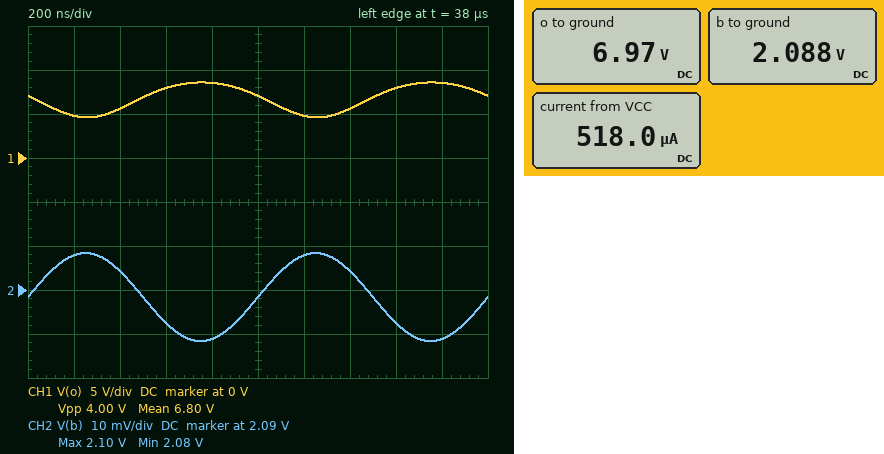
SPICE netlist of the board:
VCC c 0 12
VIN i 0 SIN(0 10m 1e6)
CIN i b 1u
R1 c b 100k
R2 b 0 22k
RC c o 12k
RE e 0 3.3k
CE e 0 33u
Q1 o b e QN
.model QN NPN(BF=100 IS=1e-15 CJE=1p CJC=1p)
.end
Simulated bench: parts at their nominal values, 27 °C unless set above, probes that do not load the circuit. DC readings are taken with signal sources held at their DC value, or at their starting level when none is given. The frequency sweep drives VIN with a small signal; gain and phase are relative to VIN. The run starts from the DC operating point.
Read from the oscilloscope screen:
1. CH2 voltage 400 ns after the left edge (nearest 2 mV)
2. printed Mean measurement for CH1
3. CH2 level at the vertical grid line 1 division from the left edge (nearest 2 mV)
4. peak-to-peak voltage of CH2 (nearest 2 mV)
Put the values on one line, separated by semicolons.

2.094 V; 6.80 V; 2.098 V; 20 mV
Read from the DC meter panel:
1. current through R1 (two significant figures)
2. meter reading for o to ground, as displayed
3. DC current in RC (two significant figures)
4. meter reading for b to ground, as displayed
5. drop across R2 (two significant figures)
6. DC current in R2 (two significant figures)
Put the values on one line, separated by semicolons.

99 µA; 6.97 V; 420 µA; 2.088 V; 2.1 V; 95 µA
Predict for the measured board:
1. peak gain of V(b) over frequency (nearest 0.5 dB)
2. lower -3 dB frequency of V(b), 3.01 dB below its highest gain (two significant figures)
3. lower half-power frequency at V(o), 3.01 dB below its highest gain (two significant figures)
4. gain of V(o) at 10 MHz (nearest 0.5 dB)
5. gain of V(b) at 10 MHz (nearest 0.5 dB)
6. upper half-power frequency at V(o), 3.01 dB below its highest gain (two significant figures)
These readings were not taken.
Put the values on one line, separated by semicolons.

0 dB; 19 Hz; 110 Hz; 45.0 dB; 0 dB; 26 MHz
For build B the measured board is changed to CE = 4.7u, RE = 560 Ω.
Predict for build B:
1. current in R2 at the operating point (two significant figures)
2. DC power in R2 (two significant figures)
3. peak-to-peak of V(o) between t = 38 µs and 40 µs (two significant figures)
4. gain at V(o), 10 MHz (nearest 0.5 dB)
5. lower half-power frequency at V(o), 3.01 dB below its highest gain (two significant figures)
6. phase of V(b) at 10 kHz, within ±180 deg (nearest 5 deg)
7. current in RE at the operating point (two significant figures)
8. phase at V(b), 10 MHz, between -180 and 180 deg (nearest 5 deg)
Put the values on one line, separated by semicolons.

58 µA; 74 µW; 3.5 V; 21.5 dB; 3.9 kHz; 15 deg; 1.0 mA; 0 deg
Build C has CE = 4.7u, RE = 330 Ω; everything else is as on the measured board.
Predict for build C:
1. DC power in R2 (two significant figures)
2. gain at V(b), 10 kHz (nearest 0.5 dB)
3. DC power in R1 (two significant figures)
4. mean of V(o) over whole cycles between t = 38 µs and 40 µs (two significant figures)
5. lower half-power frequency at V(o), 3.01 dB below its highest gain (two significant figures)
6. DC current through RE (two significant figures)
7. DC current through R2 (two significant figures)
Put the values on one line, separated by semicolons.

51 µW; -0.5 dB; 1.2 mW; 1.4 V; 4.0 kHz; 1.0 mA; 48 µA
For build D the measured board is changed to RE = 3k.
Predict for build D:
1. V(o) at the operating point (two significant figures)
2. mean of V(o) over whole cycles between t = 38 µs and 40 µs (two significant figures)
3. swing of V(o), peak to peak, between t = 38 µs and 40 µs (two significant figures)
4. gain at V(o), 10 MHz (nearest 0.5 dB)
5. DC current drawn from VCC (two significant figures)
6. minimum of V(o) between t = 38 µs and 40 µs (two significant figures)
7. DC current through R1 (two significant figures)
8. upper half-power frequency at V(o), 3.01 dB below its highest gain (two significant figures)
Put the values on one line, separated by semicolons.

6.5 V; 6.3 V; 4.3 V; 46.0 dB; 560 µA; 3.9 V; 99 µA; 25 MHz
